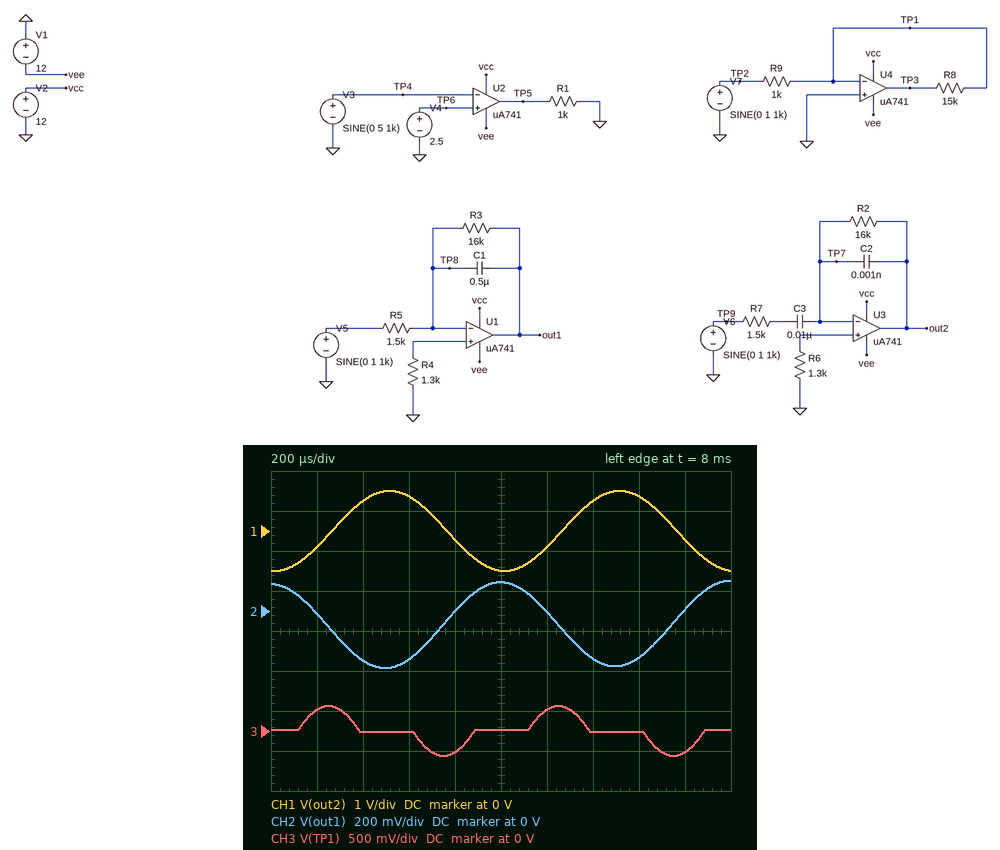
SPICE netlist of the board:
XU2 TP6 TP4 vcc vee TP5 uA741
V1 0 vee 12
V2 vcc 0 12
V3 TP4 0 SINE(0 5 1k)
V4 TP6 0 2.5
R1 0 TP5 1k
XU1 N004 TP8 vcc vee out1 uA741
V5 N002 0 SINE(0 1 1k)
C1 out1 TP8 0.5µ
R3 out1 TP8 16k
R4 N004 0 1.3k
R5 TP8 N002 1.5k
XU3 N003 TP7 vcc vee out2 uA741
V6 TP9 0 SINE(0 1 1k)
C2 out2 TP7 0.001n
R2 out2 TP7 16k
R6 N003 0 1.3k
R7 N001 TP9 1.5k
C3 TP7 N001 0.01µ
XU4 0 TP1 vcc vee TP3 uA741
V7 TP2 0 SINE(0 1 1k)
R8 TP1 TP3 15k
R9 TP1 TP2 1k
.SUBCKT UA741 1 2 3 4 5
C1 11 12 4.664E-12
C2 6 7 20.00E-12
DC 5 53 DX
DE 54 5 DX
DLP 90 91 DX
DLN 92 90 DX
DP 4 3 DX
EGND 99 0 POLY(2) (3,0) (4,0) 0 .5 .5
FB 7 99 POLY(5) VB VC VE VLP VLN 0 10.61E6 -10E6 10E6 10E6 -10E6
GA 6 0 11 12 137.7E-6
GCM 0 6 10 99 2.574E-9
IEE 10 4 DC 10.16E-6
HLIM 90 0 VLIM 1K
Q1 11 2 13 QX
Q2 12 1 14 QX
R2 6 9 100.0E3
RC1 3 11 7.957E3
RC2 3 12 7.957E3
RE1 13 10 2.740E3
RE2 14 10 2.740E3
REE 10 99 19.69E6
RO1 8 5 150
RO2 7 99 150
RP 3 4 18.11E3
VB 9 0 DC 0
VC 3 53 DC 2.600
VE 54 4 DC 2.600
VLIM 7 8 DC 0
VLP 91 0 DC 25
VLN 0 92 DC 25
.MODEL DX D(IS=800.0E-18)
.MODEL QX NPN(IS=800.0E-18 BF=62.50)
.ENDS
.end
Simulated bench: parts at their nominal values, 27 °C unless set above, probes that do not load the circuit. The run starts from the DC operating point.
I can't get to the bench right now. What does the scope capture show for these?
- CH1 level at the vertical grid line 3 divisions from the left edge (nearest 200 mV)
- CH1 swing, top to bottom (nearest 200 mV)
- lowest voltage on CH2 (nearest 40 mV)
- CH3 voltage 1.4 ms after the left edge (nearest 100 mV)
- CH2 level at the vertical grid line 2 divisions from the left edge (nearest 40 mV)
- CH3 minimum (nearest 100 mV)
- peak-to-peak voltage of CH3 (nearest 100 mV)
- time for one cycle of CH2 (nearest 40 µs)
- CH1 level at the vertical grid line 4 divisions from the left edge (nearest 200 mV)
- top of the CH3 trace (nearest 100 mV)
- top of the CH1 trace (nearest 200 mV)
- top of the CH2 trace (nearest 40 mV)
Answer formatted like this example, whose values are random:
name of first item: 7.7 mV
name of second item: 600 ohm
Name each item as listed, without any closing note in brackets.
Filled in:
CH1 level at the vertical grid line 3 divisions from the left edge: 800 mV
CH1 swing, top to bottom: 2.0 V
lowest voltage on CH2: -280 mV
CH3 voltage 1.4 ms after the left edge: 0 V
CH2 level at the vertical grid line 2 divisions from the left edge: -240 mV
CH3 minimum: -300 mV
peak-to-peak voltage of CH3: 600 mV
time for one cycle of CH2: 1.00 ms
CH1 level at the vertical grid line 4 divisions from the left edge: -200 mV
top of the CH3 trace: 300 mV
top of the CH1 trace: 1.0 V
top of the CH2 trace: 160 mV
